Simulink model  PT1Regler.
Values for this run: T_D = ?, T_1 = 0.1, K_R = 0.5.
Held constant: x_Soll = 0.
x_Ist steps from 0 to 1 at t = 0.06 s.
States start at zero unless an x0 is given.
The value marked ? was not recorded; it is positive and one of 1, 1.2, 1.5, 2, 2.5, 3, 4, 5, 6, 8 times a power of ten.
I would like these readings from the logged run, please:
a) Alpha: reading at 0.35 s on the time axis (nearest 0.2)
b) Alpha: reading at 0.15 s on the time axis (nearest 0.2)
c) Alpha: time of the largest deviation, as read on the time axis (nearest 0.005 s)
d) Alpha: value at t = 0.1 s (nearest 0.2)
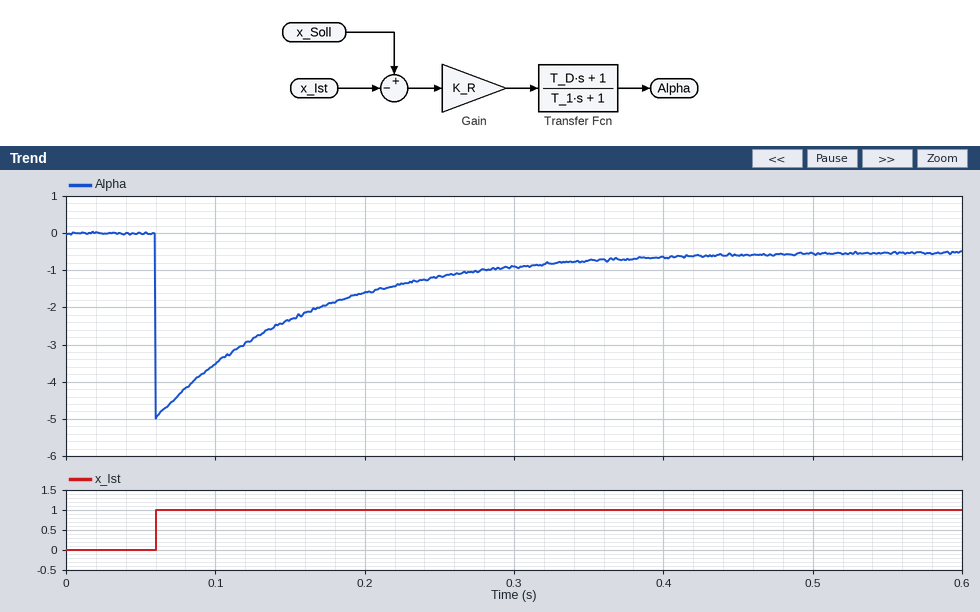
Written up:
-0.8
-2.4
0.060 s
-3.6
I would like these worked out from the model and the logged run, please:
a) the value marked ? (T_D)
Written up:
1
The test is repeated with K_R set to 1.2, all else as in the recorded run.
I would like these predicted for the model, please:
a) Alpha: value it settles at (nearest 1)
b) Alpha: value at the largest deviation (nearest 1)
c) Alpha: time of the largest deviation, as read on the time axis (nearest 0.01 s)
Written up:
-1
-12
0.06 s
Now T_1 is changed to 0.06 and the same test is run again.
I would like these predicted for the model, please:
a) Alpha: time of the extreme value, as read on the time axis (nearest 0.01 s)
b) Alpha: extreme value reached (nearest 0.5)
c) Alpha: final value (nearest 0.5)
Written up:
0.06 s
-8.5
-0.5
